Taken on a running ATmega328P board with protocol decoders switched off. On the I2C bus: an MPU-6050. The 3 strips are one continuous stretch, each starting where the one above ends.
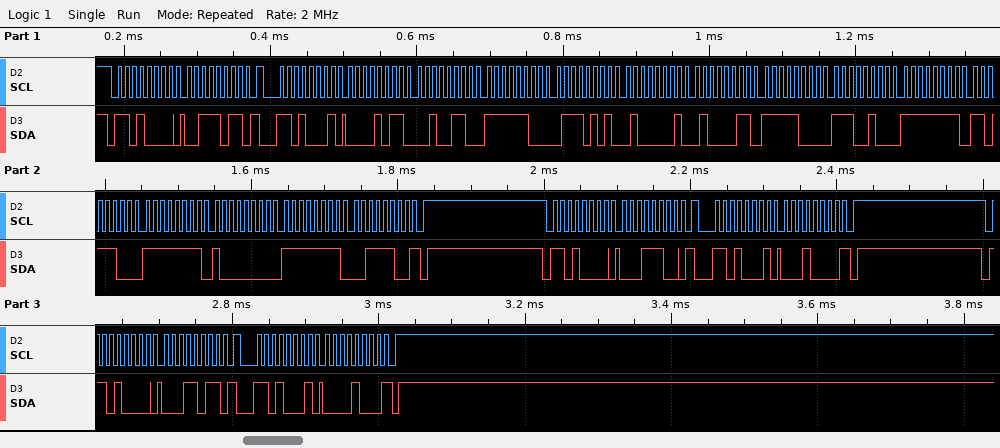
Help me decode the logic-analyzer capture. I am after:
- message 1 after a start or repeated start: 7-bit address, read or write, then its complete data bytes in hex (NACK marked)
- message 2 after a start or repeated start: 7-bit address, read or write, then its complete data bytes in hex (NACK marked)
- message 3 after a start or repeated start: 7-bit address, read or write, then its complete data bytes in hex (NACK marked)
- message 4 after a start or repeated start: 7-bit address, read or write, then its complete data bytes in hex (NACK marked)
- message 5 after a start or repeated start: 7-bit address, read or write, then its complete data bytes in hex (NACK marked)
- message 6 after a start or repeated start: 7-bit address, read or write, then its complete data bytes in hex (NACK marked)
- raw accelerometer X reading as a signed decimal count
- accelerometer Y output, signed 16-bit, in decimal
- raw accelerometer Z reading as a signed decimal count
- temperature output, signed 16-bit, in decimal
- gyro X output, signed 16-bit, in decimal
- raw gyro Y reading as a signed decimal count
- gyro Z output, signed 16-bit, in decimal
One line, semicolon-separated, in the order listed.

0x68 write: 3B; 0x68 read: 0B 26 FC 75 41 43 F8 E4 FF DC FF 80 FF 3C NACK; 0x68 write: 1C; 0x68 read: 10 NACK; 0x68 write: 1B; 0x68 read: 08 NACK; 2854; -907; 16707; -1820; -36; -128; -196
